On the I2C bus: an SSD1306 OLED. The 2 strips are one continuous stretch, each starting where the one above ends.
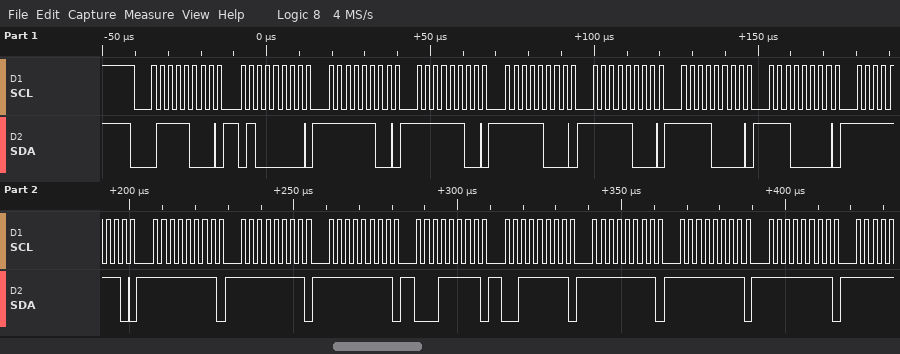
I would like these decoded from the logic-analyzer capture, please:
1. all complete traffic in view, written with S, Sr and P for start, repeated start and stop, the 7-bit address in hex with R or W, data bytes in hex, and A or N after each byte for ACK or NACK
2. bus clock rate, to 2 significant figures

S 3CW A 40 A FC A FC A F8 A F8 A F0 A E0 A FE A FF A FF A FF A 1F A 3F A FF A FF A FF A
400 kHz
